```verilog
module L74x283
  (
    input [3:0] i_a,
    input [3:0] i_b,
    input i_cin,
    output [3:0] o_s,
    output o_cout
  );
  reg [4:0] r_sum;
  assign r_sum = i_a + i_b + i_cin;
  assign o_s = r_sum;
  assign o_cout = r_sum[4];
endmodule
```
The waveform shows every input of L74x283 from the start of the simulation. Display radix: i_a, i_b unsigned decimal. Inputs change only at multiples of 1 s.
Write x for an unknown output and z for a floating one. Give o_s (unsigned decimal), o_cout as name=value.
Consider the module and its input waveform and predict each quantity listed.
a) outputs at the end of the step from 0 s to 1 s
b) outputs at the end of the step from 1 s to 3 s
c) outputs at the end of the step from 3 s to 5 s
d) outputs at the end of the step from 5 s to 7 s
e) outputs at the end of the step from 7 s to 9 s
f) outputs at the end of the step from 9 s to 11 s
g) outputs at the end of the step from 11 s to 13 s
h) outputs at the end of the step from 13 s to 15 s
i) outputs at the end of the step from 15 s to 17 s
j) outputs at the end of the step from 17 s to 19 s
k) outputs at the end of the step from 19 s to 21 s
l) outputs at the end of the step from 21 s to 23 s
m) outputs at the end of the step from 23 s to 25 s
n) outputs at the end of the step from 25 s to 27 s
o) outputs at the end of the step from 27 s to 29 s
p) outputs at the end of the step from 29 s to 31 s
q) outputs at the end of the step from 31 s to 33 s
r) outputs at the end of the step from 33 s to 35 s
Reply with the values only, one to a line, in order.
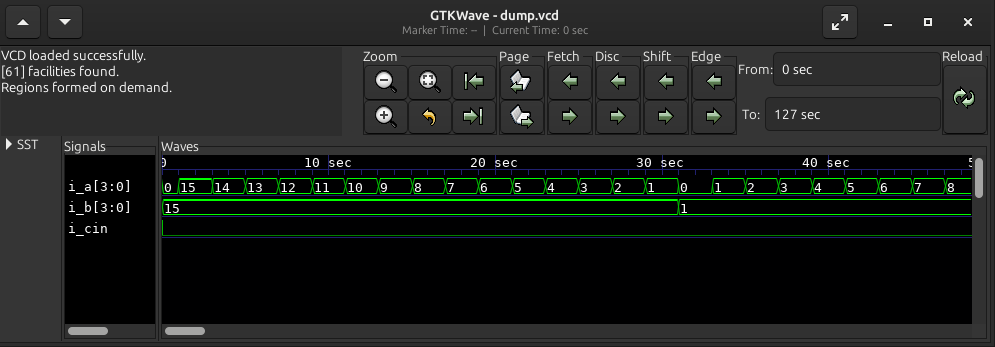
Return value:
o_s=15, o_cout=0
o_s=14, o_cout=1
o_s=13, o_cout=1
o_s=12, o_cout=1
o_s=11, o_cout=1
o_s=10, o_cout=1
o_s=9, o_cout=1
o_s=8, o_cout=1
o_s=7, o_cout=1
o_s=6, o_cout=1
o_s=5, o_cout=1
o_s=4, o_cout=1
o_s=3, o_cout=1
o_s=2, o_cout=1
o_s=1, o_cout=1
o_s=0, o_cout=1
o_s=1, o_cout=0
o_s=2, o_cout=0
